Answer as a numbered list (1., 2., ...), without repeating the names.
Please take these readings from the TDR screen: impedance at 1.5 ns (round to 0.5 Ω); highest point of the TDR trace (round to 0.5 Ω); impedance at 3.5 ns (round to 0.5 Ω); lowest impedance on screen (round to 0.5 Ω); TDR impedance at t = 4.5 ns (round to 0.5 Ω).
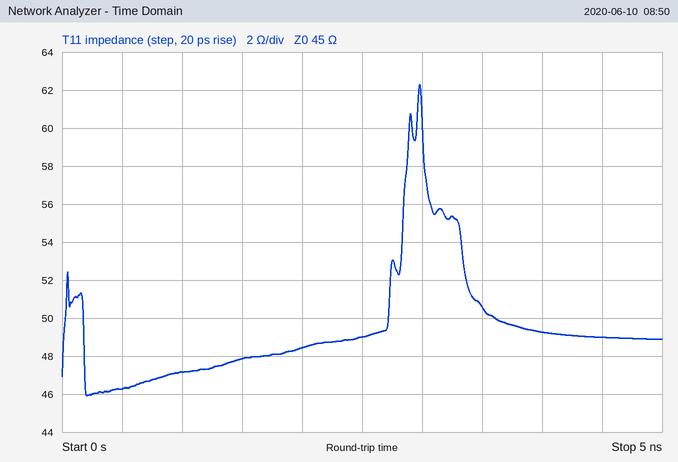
1. 48.0 Ω
2. 62.5 Ω
3. 50.5 Ω
4. 46.0 Ω
5. 49.0 Ω
